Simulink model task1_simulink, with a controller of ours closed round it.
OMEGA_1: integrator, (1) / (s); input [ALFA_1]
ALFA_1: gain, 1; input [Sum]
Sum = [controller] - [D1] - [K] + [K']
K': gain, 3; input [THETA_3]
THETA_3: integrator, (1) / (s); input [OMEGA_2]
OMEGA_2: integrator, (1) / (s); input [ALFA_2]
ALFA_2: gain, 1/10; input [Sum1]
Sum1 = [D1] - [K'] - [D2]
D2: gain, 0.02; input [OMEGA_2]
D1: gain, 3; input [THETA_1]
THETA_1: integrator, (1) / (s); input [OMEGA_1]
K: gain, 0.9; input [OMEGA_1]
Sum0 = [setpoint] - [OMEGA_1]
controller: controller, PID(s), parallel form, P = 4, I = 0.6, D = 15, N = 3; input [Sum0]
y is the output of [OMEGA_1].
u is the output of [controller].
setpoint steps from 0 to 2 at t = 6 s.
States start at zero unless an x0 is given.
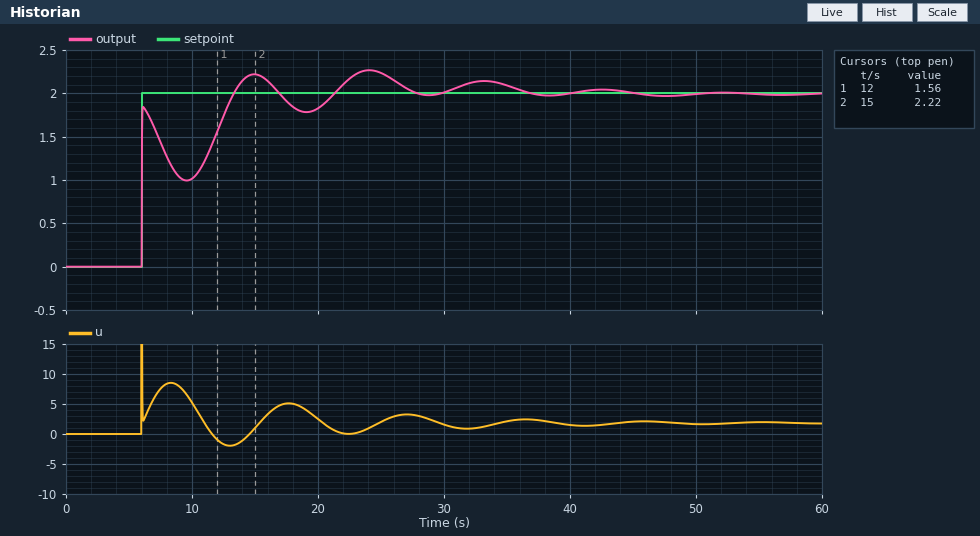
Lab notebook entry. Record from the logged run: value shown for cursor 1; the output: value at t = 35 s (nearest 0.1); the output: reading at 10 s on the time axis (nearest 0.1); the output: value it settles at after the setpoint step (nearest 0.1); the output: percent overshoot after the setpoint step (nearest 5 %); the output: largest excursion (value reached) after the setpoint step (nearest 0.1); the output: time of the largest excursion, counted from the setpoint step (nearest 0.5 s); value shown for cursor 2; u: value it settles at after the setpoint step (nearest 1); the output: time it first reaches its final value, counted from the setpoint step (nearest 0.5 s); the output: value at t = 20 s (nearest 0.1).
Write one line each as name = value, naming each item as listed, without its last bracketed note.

value shown for cursor 1 = 1.56
the output: value at t = 35 s = 2.1
the output: reading at 10 s on the time axis = 1.0
the output: value it settles at after the setpoint step = 2.0
the output: percent overshoot after the setpoint step = 15 %
the output: largest excursion (value reached) after the setpoint step = 2.3
the output: time of the largest excursion, counted from the setpoint step = 18.0 s
value shown for cursor 2 = 2.22
u: value it settles at after the setpoint step = 2
the output: time it first reaches its final value, counted from the setpoint step = 7.5 s
the output: value at t = 20 s = 1.8
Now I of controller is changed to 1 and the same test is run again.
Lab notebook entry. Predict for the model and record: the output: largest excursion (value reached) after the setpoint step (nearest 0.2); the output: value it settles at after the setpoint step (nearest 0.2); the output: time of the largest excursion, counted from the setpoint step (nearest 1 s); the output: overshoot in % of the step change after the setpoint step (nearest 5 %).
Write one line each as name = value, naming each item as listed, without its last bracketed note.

the output: largest excursion (value reached) after the setpoint step = 2.4
the output: value it settles at after the setpoint step = 2.0
the output: time of the largest excursion, counted from the setpoint step = 9 s
the output: overshoot in % of the step change after the setpoint step = 20 %
